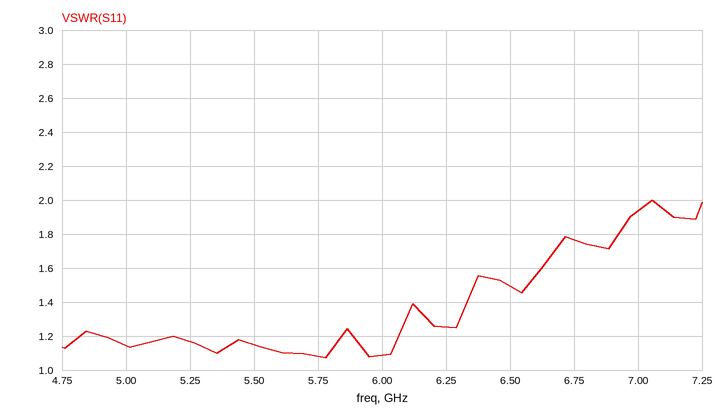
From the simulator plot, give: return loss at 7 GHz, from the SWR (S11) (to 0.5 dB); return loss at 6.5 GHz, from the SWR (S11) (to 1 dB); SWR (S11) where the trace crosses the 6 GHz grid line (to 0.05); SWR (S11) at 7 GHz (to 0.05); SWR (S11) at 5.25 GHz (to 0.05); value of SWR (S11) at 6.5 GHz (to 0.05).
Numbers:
10.0 dB
14 dB
1.10
1.95
1.15
1.50
